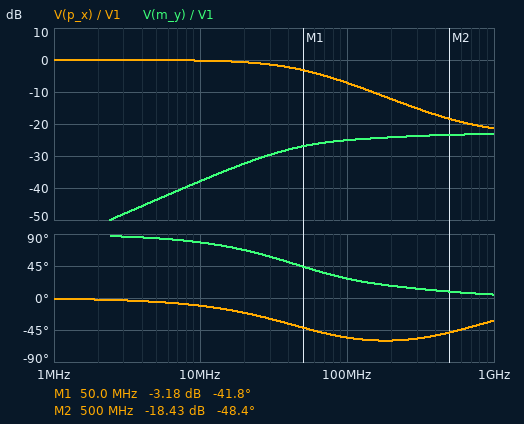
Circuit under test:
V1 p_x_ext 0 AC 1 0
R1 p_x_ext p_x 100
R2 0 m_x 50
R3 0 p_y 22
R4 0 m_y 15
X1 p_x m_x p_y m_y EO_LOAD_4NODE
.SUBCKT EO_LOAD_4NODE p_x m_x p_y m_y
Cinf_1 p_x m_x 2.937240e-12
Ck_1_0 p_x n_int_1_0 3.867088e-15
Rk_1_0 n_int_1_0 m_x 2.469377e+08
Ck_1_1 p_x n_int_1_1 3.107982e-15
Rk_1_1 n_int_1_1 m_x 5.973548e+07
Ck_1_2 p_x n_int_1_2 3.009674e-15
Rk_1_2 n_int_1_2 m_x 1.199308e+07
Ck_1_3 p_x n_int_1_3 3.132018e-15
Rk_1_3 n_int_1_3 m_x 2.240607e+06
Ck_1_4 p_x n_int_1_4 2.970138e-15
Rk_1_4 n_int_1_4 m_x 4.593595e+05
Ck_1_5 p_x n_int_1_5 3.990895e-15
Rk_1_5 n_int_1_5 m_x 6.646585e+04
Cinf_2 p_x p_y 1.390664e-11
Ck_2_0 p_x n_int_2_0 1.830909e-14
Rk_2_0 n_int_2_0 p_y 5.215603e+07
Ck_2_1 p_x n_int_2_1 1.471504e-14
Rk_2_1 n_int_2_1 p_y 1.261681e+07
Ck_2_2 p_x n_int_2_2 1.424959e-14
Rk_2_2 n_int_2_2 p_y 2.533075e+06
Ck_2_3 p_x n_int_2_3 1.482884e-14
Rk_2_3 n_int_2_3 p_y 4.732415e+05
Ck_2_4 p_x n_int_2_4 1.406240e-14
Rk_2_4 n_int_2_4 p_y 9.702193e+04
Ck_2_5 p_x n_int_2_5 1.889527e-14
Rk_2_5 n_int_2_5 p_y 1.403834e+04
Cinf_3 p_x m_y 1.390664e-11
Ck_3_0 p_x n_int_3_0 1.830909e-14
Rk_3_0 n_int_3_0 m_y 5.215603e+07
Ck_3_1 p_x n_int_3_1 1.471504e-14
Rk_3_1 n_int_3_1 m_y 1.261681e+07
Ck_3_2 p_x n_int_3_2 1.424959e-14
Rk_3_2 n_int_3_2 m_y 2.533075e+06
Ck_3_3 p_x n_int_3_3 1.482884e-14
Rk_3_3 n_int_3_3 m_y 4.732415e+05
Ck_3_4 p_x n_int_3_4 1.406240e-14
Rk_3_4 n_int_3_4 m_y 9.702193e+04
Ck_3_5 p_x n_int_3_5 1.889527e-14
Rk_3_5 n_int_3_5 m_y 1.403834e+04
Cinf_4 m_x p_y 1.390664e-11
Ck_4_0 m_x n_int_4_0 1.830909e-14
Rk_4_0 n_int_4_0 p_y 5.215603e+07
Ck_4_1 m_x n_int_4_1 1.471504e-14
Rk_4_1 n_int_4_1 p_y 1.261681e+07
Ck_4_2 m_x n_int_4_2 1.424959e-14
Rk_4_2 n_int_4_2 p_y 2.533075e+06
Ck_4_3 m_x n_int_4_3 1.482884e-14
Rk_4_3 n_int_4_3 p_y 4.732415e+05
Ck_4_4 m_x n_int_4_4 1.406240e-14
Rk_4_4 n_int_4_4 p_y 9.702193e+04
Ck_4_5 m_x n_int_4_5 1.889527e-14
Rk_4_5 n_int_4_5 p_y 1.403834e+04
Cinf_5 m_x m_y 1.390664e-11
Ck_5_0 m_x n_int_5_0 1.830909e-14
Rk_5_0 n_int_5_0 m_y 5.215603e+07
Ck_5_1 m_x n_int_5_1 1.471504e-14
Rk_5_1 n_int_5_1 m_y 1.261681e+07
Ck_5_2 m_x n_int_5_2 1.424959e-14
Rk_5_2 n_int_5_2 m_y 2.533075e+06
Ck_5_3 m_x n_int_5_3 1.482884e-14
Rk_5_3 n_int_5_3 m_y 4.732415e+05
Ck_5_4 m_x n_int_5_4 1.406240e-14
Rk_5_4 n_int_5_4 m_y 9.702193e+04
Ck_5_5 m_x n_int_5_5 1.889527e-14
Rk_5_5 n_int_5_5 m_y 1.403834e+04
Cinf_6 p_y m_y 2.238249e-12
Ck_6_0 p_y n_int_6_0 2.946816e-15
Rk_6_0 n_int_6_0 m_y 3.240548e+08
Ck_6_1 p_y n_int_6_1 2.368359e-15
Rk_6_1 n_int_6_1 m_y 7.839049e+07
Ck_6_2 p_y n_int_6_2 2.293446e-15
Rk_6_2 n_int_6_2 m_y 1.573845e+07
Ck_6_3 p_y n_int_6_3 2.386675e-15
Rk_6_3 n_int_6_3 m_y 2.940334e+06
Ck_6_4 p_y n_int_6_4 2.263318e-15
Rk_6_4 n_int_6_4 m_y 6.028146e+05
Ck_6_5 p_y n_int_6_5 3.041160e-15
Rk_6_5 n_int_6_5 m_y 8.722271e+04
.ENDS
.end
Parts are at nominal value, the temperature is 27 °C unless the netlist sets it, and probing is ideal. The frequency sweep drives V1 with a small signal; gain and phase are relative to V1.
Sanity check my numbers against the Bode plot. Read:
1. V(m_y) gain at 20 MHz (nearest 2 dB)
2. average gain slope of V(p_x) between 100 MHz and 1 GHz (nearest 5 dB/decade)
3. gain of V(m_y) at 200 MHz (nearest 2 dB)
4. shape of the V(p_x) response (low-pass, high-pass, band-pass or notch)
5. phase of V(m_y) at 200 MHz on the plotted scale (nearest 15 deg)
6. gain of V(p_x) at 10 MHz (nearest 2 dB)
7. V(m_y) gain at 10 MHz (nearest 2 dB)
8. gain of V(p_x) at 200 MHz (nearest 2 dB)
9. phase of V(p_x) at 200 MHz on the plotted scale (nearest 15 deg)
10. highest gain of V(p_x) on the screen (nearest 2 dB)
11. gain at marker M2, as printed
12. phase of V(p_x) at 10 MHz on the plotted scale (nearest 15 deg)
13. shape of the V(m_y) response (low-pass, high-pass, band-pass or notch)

-32 dB
-15 dB/decade
-24 dB
low-pass
15 deg
0 dB
-38 dB
-12 dB
-60 deg
0 dB
-18.43 dB
-15 deg
high-pass
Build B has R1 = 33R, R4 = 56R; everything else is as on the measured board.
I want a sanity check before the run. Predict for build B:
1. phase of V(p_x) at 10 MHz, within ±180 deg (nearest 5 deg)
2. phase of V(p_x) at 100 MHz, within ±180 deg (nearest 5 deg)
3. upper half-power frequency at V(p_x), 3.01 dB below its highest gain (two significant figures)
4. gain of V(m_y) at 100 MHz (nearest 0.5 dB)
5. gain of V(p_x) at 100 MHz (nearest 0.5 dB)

-5 deg
-25 deg
130 MHz
-11.5 dB
-2.0 dB
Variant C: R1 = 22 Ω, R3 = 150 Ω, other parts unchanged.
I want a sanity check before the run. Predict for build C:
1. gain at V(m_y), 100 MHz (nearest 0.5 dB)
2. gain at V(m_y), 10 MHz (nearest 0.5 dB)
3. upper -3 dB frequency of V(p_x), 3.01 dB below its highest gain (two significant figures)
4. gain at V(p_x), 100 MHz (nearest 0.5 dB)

-18.0 dB
-37.5 dB
210 MHz
-1.0 dB
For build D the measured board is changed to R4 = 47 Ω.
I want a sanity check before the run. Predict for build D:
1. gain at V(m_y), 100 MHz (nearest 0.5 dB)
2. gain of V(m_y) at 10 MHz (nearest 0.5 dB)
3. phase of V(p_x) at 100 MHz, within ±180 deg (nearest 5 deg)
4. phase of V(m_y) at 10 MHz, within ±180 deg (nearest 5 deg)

-17.5 dB
-28.0 dB
-50 deg
75 deg
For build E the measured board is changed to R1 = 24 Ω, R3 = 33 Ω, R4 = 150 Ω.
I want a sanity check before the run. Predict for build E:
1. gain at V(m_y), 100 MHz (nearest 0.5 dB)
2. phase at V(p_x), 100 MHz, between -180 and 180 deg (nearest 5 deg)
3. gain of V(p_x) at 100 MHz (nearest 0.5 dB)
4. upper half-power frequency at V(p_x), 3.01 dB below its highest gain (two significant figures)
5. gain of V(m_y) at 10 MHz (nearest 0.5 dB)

-8.0 dB
-20 deg
-1.5 dB
180 MHz
-18.0 dB
